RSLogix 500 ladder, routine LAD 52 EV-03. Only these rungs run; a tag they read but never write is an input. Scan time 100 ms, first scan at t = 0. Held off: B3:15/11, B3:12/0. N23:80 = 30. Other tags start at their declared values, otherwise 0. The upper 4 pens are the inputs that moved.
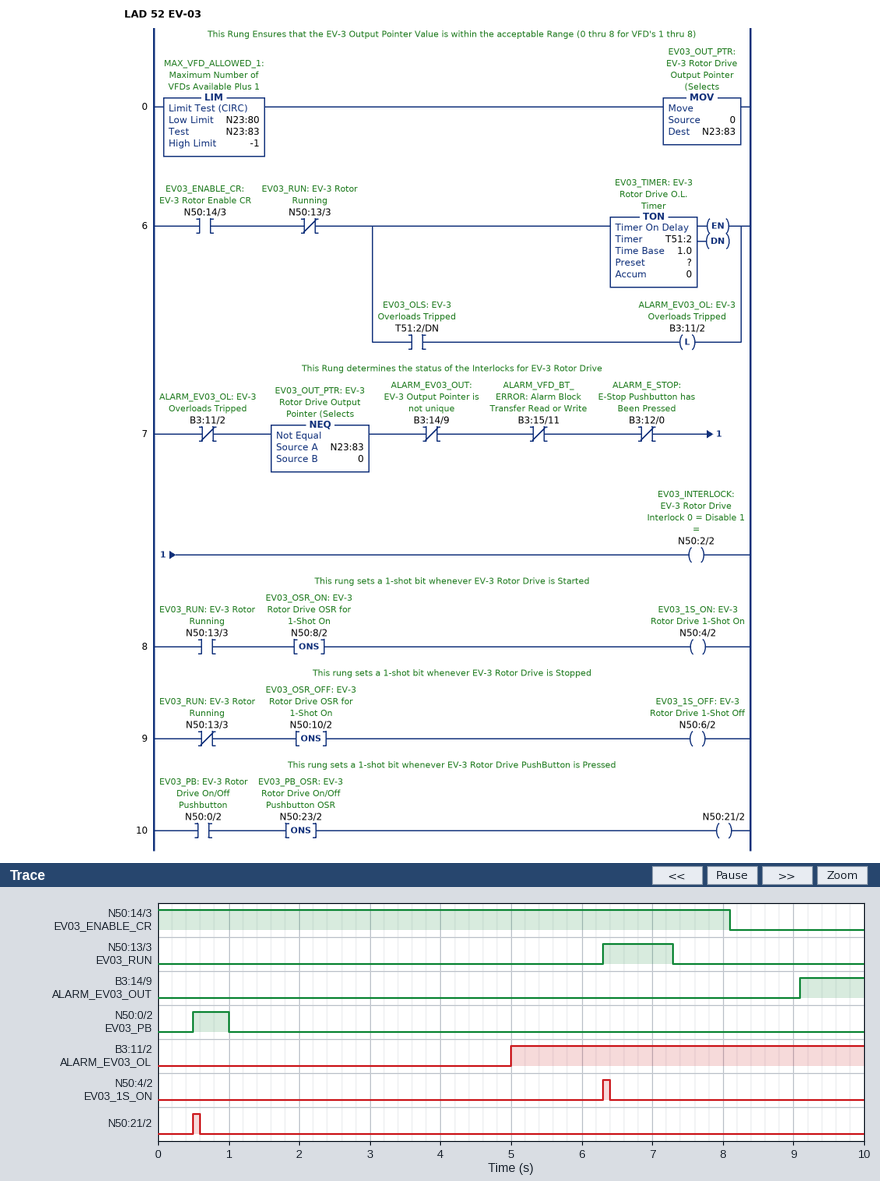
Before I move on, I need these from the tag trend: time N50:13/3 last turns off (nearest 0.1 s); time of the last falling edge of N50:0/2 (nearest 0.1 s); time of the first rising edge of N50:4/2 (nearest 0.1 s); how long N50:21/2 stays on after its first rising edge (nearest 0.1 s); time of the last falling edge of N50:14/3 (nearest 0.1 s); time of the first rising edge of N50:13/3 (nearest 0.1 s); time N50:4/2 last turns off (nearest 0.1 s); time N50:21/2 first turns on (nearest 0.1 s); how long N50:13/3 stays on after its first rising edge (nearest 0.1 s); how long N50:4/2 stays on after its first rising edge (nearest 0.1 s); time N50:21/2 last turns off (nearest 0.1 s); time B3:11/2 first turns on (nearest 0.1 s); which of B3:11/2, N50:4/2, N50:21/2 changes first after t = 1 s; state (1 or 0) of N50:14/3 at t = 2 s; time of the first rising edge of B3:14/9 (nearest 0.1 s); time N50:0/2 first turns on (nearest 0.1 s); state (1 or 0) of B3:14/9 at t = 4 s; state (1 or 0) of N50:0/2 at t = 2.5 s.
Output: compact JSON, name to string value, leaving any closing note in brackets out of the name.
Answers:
{"time N50:13/3 last turns off": "7.3 s", "time of the last falling edge of N50:0/2": "1.0 s", "time of the first rising edge of N50:4/2": "6.3 s", "how long N50:21/2 stays on after its first rising edge": "0.1 s", "time of the last falling edge of N50:14/3": "8.1 s", "time of the first rising edge of N50:13/3": "6.3 s", "time N50:4/2 last turns off": "6.4 s", "time N50:21/2 first turns on": "0.5 s", "how long N50:13/3 stays on after its first rising edge": "1.0 s", "how long N50:4/2 stays on after its first rising edge": "0.1 s", "time N50:21/2 last turns off": "0.6 s", "time B3:11/2 first turns on": "5.0 s", "which of B3:11/2, N50:4/2, N50:21/2 changes first after t = 1 s": "B3:11/2", "state (1 or 0) of N50:14/3 at t = 2 s": "1", "time of the first rising edge of B3:14/9": "9.1 s", "time N50:0/2 first turns on": "0.5 s", "state (1 or 0) of B3:14/9 at t = 4 s": "0", "state (1 or 0) of N50:0/2 at t = 2.5 s": "0"}
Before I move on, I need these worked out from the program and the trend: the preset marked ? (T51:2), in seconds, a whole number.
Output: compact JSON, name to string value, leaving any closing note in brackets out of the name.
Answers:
{"the preset marked ? (T51:2), in seconds, a whole number": "5 s"}
